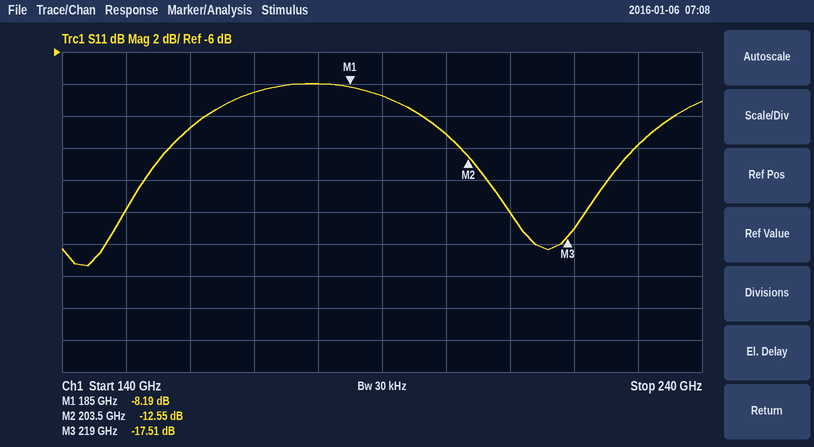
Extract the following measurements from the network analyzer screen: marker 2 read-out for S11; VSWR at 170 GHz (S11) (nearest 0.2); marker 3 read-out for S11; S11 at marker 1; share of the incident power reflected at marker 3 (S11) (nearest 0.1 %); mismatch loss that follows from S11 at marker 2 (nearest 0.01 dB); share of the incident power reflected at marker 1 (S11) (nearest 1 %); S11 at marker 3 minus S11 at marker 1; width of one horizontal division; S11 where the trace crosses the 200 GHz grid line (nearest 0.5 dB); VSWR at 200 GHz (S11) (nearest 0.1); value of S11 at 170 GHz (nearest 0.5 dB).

-12.55 dB
2.2
-17.51 dB
-8.19 dB
1.8 %
0.25 dB
15 %
-9.32 dB
10 GHz
-11.0 dB
1.8
-8.5 dB
